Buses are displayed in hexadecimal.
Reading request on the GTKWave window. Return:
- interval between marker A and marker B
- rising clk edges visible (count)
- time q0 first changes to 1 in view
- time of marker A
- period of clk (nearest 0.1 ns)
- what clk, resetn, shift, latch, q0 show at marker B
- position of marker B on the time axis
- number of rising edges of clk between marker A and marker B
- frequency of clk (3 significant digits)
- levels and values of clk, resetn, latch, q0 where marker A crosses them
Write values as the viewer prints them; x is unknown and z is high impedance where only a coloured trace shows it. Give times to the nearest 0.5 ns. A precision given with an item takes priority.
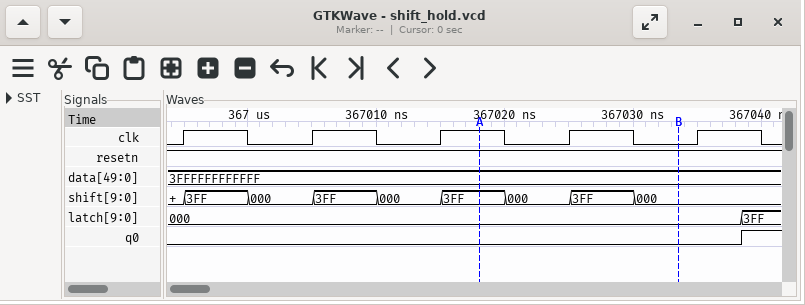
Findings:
15.5 ns
5
367038.5 ns
367018 ns
10 ns
clk=0, resetn=1, shift=000, latch=000, q0=0
367033.5 ns
1
100 MHz
clk=1, resetn=1, latch=000, q0=0
